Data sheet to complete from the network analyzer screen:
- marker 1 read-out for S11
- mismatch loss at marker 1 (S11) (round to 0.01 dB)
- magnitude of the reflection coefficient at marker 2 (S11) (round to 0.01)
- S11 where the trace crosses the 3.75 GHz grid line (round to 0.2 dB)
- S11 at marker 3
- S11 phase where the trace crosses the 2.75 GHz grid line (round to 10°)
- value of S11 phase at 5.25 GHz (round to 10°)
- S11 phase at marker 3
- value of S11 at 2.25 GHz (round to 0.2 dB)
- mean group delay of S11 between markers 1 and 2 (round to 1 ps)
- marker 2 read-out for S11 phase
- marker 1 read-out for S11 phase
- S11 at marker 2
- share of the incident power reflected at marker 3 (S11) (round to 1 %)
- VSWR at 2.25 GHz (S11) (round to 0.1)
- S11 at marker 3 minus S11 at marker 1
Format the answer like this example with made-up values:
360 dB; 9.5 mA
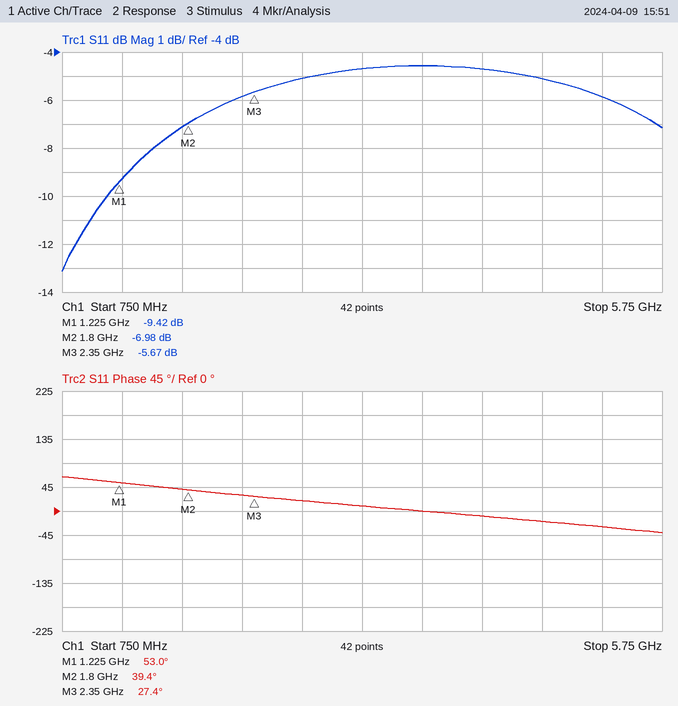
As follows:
-9.42 dB; 0.53 dB; 0.45; -4.6 dB; -5.67 dB; 20°; -30°; 27.4°; -5.8 dB; 66 ps; 39.4°; 53.0°; -6.98 dB; 27 %; 3.1; 3.75 dB
